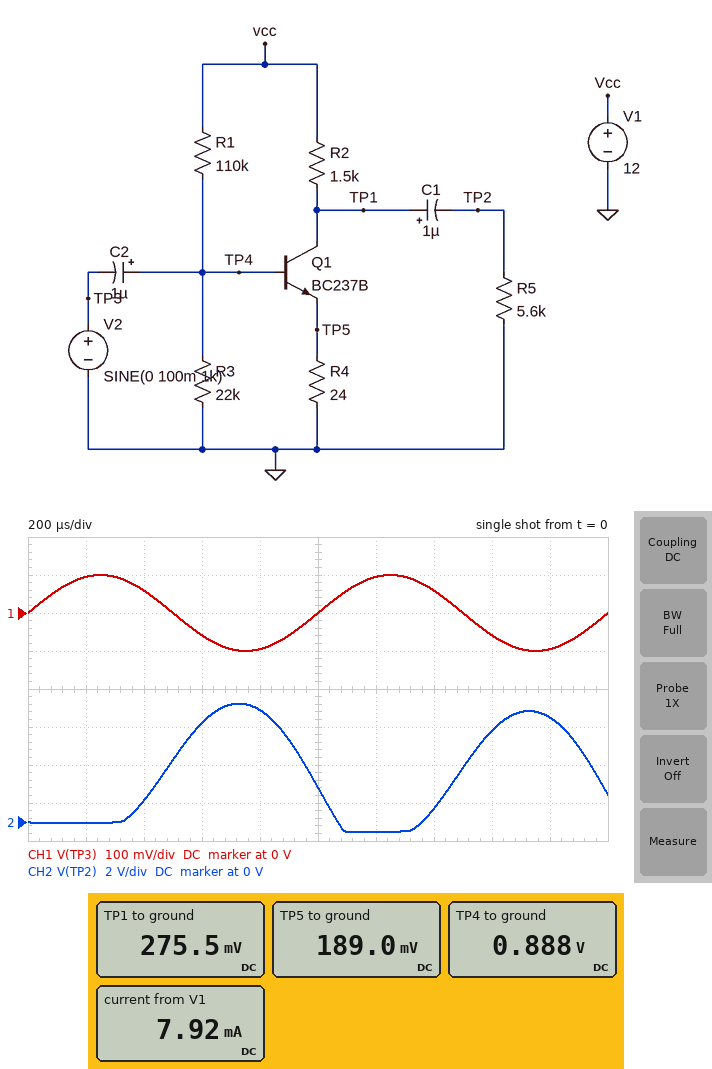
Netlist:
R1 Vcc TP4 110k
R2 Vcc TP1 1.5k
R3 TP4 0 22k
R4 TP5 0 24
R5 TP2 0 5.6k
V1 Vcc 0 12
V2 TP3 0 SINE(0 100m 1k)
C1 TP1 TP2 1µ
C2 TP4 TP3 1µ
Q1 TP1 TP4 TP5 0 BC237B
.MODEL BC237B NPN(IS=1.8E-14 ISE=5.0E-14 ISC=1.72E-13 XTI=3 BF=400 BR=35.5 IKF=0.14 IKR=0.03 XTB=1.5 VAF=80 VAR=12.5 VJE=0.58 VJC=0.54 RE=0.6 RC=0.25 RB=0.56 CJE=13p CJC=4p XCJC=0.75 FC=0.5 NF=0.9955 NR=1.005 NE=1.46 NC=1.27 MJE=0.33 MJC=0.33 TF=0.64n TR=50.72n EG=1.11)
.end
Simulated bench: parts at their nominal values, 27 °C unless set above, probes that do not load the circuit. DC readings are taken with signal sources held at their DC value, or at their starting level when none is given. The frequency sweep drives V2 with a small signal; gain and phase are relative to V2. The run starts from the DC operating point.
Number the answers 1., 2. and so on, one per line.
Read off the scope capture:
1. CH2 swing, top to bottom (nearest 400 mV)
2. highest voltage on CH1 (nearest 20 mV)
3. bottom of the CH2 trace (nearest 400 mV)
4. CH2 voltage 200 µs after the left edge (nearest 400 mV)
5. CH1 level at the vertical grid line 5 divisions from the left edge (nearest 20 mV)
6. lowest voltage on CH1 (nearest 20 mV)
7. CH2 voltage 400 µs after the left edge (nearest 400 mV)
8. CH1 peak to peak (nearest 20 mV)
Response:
1. 6.8 V
2. 100 mV
3. -400 mV
4. 0 V
5. 0 V
6. -100 mV
7. 1.2 V
8. 200 mV
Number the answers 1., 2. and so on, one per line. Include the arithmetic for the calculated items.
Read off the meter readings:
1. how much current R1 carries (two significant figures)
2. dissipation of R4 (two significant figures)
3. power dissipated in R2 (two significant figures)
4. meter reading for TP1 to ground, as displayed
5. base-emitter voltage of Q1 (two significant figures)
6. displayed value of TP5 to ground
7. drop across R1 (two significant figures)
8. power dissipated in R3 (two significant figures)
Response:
1. (12 V - 888 mV) / 110 kΩ = 100 µA
2. (189 mV)^2 / 24 Ω = 1.5 mW
3. (12 V - 275.5 mV)^2 / 1.5 kΩ = 92 mW
4. 275.5 mV
5. 888 mV - 189 mV = 700 mV
6. 189.0 mV
7. 12 V - 888 mV = 11 V
8. (888 mV)^2 / 22 kΩ = 36 µW
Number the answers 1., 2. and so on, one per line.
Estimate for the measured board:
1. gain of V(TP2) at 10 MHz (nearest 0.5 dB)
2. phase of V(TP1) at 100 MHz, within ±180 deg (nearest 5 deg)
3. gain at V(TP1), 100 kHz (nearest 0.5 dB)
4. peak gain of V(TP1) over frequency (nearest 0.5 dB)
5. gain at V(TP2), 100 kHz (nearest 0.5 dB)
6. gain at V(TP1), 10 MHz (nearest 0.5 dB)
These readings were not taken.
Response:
1. 2.0 dB
2. 5 deg
3. 19.0 dB
4. 19.0 dB
5. 19.0 dB
6. 2.0 dB
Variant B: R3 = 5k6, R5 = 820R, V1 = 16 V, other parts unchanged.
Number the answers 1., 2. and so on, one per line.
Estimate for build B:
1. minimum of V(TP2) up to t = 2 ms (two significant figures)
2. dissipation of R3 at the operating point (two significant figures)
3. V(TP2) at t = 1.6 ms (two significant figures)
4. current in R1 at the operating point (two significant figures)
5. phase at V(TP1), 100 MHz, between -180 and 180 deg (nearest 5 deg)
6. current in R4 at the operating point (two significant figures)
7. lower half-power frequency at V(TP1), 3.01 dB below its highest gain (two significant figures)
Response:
1. -1.5 V
2. 95 µW
3. 1.0 V
4. 140 µA
5. 130 deg
6. 2.8 mA
7. 24 Hz
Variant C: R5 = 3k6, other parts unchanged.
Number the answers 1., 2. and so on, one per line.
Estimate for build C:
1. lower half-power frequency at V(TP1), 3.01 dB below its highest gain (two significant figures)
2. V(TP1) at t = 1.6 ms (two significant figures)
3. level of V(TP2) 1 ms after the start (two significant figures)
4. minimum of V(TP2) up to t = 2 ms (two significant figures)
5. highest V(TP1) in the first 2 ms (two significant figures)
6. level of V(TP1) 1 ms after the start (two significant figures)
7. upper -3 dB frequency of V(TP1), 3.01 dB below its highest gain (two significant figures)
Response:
1. 1.7 kHz
2. 5.1 V
3. 1.5 V
4. -700 mV
5. 6.2 V
6. 2.4 V
7. 900 kHz
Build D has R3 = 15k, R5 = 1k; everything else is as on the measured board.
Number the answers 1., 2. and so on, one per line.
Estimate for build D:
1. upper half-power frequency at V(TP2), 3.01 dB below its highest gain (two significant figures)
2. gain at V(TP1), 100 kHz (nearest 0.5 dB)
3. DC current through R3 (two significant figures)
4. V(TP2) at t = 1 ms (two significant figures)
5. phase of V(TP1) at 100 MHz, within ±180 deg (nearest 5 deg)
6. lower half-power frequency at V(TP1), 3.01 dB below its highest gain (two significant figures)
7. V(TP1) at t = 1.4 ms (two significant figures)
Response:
1. 1.7 MHz
2. 21.5 dB
3. 59 µA
4. 800 mV
5. 10 deg
6. 990 Hz
7. 1.0 V
